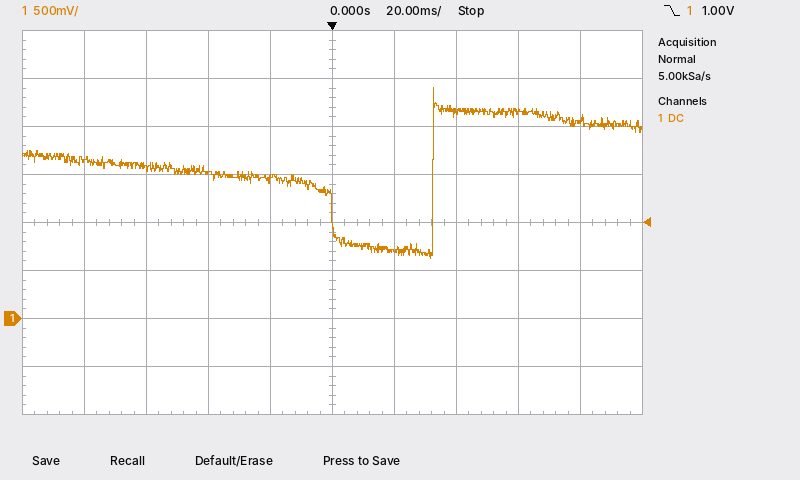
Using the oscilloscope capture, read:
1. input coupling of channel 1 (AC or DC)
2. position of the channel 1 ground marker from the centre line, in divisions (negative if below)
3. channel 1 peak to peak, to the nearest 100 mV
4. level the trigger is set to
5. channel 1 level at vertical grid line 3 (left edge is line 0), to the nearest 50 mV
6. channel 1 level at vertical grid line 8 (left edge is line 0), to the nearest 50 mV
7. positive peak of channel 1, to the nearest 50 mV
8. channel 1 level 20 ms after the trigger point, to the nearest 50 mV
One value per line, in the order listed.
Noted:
DC
-2.0 div
1.80 V
1.00 V
1.50 V
2.15 V
2.40 V
700 mV
